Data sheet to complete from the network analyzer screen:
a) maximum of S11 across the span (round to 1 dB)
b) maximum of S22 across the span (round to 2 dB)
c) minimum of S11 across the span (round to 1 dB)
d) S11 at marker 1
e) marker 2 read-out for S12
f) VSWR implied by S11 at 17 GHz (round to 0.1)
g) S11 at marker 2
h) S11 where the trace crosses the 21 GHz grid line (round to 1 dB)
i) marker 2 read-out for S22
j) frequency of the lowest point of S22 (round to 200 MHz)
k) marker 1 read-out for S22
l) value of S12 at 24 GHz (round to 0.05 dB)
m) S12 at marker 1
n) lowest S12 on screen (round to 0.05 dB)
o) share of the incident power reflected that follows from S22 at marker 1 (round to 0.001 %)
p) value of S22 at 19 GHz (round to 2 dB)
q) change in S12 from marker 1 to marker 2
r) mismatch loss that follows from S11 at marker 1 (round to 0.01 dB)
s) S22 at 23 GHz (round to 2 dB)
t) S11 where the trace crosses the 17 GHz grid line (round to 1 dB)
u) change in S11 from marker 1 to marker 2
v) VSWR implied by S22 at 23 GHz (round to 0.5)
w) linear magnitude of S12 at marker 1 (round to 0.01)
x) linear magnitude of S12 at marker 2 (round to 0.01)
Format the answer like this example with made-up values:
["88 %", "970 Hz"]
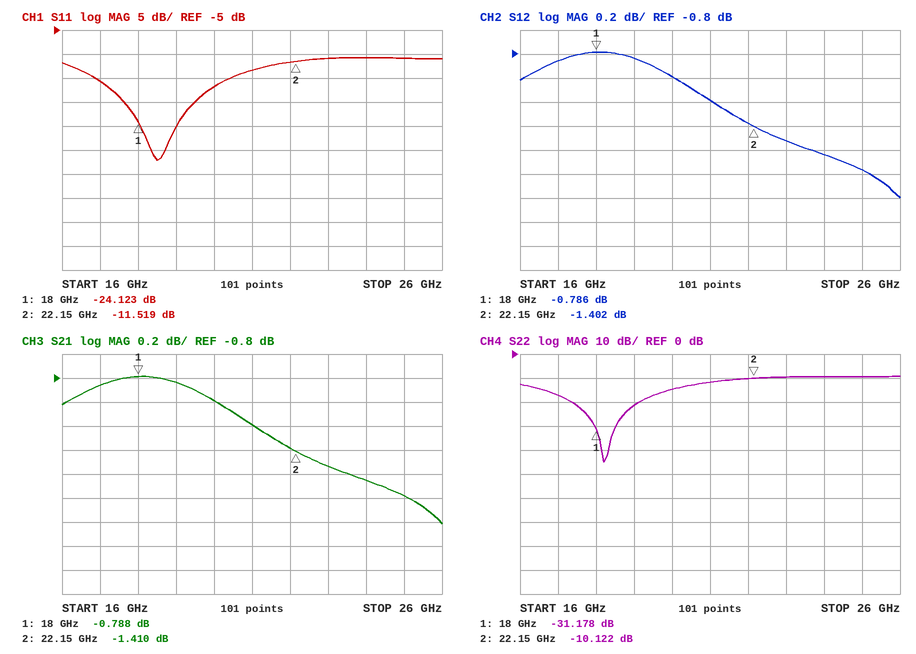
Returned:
["-11 dB", "-10 dB", "-32 dB", "-24.123 dB", "-1.402 dB", "1.4", "-11.519 dB", "-13 dB", "-10.122 dB", "18.2 GHz", "-31.178 dB", "-1.65 dB", "-0.786 dB", "-2.00 dB", "0.076 %", "-22 dB", "-0.616 dB", "0.02 dB", "-10 dB", "-16 dB", "12.604 dB", "2.0", "0.91", "0.85"]
